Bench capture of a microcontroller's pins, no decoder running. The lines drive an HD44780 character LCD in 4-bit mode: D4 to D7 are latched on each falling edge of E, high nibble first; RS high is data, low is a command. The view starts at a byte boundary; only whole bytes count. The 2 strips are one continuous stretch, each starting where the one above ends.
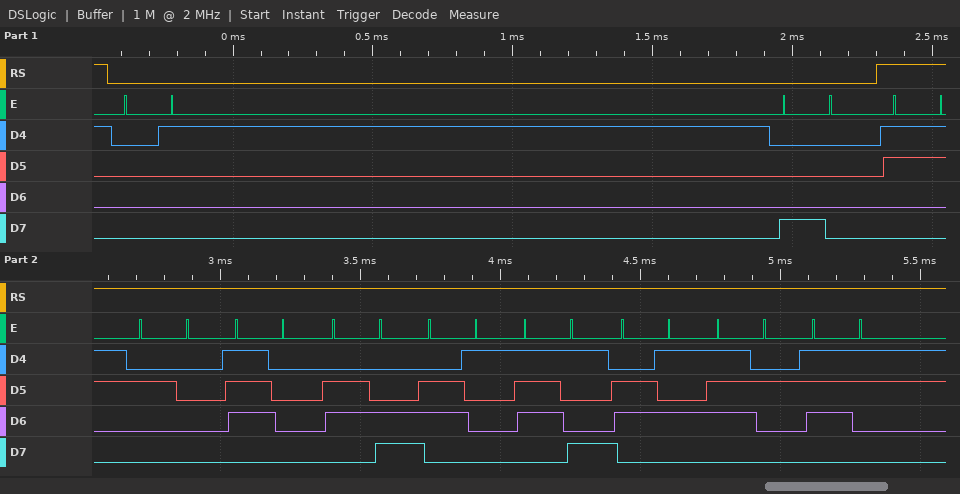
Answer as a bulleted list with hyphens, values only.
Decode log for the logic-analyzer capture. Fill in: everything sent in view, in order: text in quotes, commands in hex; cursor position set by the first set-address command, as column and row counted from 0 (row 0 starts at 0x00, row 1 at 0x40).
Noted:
- 0x01 0x80 "3 players"
- column 0, row 0
